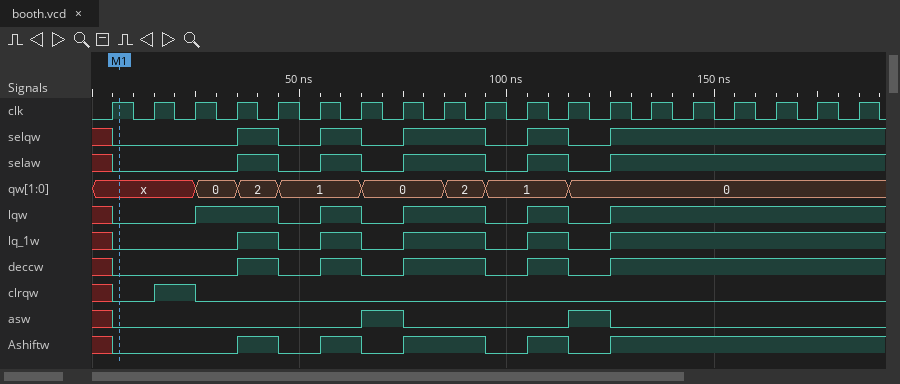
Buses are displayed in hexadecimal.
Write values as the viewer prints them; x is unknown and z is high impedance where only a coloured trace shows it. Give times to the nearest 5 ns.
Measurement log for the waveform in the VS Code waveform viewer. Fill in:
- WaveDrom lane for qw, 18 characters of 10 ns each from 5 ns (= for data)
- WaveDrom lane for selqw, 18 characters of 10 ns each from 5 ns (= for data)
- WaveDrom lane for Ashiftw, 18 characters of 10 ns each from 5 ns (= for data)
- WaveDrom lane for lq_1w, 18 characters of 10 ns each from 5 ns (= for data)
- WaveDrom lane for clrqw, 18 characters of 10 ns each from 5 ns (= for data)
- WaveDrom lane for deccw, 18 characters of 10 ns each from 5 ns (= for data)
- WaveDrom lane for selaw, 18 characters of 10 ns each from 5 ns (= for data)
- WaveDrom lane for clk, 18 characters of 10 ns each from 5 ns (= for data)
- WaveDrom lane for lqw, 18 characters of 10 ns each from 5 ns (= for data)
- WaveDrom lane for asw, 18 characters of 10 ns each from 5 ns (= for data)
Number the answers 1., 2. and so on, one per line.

1. {name: 'qw', wave: 'x.===.=.==.=......', data: '0 2 1 0 2 1 0'}
2. {name: 'selqw', wave: '0..10101.0101.....'}
3. {name: 'Ashiftw', wave: '0..10101.0101.....'}
4. {name: 'lq_1w', wave: '0..10101.0101.....'}
5. {name: 'clrqw', wave: '010...............'}
6. {name: 'deccw', wave: '0..10101.0101.....'}
7. {name: 'selaw', wave: '0..10101.0101.....'}
8. {name: 'clk', wave: 'p.................'}
9. {name: 'lqw', wave: '0.1.0101.0101.....'}
10. {name: 'asw', wave: '0.....10...10.....'}
